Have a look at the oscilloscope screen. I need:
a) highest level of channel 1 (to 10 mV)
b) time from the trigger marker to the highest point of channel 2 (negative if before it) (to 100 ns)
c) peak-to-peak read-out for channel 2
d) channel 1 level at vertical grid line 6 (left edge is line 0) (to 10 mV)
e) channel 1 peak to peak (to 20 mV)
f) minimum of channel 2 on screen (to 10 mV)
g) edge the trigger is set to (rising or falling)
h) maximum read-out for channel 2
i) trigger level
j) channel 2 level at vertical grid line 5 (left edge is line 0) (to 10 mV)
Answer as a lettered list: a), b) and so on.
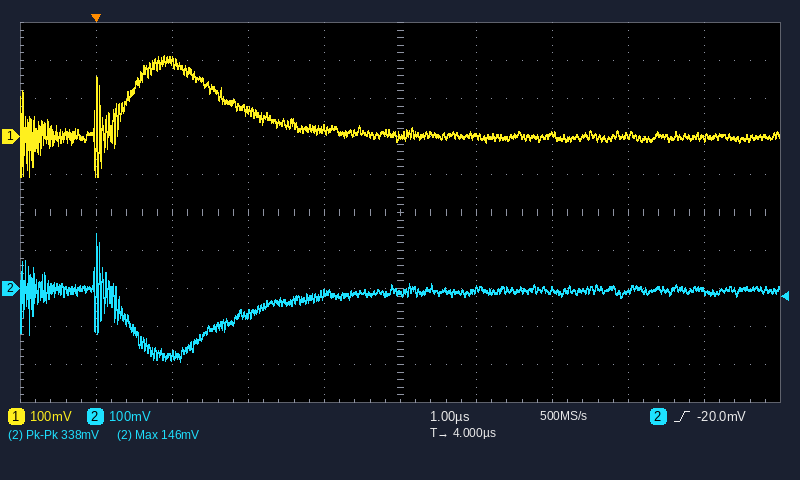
a) 210 mV
b) 0.0 µs
c) 338 mV
d) 0 mV
e) 320 mV
f) -190 mV
g) rising
h) 146 mV
i) -20.0 mV
j) -10 mV
